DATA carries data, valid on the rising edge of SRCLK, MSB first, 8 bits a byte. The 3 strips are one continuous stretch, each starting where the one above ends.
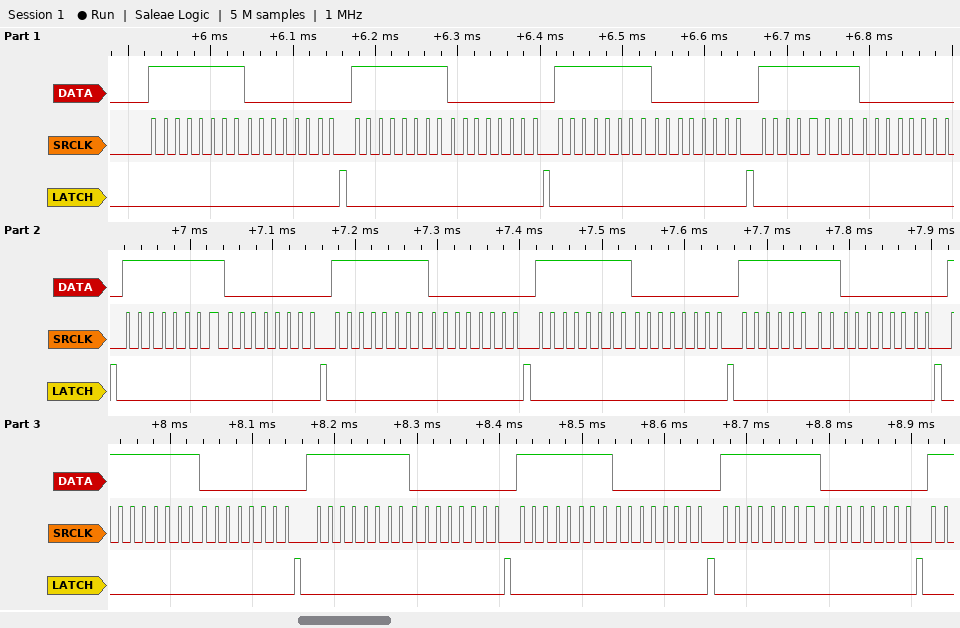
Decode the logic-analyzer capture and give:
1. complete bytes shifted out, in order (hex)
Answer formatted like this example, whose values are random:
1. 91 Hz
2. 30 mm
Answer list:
1. FF 00 FF 00 FF 00 FF 00 FF 00 FF 00 FF 00 FF 00 FF 00 FF 00 FF 00 FF 00
